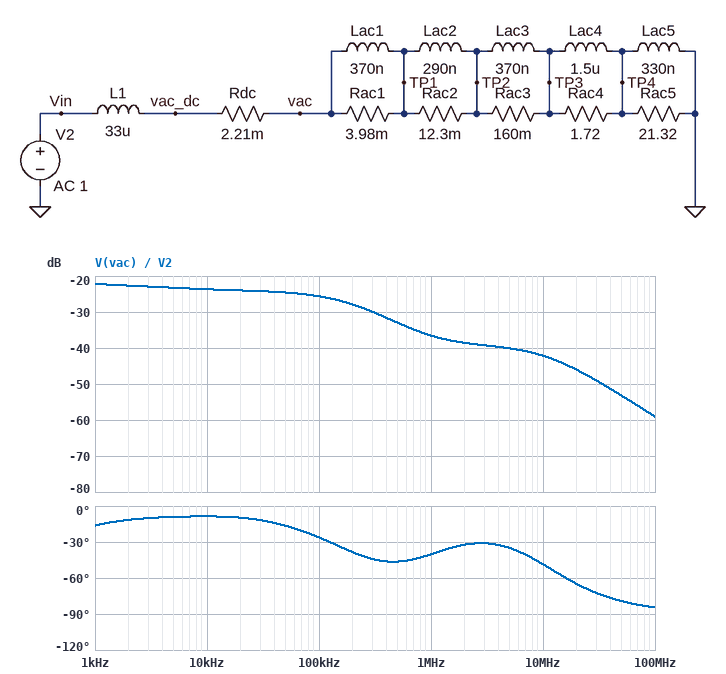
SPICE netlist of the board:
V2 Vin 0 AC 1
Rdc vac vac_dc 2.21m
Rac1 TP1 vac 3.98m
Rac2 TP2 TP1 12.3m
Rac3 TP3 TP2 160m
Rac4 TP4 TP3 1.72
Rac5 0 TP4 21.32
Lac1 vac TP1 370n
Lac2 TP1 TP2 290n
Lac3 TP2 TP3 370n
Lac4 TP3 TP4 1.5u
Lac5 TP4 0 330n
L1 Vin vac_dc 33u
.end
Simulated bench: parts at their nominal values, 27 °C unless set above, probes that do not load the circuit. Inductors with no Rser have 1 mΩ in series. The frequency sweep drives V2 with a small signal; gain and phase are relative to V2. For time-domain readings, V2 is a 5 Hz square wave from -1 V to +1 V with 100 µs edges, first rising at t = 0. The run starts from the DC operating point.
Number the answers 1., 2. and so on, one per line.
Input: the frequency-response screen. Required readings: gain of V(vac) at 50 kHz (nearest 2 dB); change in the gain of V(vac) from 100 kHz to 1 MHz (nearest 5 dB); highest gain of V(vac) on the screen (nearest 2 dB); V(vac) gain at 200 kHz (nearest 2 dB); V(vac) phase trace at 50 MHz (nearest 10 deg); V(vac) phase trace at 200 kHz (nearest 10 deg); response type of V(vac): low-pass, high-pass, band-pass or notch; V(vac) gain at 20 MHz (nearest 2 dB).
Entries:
1. -24 dB
2. -10 dB
3. -22 dB
4. -28 dB
5. -80 deg
6. -40 deg
7. low-pass
8. -46 dB
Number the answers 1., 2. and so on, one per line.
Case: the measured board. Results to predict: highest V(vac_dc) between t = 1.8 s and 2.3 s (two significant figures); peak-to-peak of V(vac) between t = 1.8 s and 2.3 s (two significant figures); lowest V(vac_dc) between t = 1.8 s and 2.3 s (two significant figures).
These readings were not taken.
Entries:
1. 870 mV
2. 1.2 V
3. -870 mV
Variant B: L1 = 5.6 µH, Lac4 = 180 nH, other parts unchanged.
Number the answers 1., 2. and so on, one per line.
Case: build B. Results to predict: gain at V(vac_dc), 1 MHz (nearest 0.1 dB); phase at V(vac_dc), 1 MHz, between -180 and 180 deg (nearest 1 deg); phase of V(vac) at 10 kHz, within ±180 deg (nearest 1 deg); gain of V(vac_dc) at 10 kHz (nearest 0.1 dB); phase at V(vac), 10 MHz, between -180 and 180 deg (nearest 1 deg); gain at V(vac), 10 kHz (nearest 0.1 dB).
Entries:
1. -22.1 dB
2. -16 deg
3. -14 deg
4. -16.2 dB
5. -46 deg
6. -16.3 dB
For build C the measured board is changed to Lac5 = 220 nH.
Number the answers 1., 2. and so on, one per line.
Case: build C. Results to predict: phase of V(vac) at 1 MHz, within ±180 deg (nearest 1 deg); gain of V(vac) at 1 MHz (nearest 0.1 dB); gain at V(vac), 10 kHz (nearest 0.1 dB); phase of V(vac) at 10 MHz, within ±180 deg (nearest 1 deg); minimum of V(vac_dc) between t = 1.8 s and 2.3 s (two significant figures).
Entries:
1. -48 deg
2. -38.2 dB
3. -24.1 dB
4. -40 deg
5. -870 mV
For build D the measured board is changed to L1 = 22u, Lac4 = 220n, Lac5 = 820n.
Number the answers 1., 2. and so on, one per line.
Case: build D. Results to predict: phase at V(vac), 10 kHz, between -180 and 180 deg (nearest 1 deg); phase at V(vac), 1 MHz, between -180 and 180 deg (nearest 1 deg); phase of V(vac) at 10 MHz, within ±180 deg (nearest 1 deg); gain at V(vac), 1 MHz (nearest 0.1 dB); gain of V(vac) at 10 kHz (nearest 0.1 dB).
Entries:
1. -10 deg
2. -19 deg
3. -68 deg
4. -27.5 dB
5. -23.8 dB
